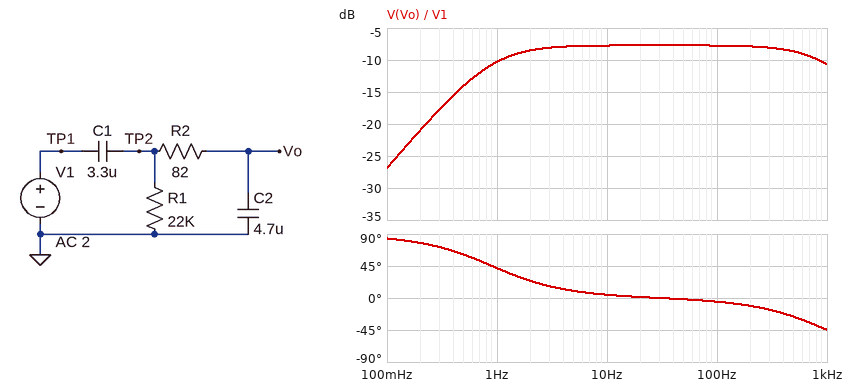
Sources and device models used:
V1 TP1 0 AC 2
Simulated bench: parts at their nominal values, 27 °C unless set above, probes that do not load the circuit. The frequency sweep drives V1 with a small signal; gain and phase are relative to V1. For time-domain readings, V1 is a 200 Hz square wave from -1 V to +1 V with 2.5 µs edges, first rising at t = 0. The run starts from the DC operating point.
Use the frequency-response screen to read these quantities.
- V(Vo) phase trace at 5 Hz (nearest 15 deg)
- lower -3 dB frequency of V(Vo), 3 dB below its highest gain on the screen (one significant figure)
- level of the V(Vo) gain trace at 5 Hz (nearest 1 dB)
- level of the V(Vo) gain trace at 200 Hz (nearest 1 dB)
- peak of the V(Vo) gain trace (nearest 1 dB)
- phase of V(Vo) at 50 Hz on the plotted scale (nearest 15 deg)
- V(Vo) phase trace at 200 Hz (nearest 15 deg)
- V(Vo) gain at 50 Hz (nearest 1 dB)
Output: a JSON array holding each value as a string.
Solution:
["15 deg", "900 mHz", "-8 dB", "-8 dB", "-8 dB", "0 deg", "-15 deg", "-8 dB"]
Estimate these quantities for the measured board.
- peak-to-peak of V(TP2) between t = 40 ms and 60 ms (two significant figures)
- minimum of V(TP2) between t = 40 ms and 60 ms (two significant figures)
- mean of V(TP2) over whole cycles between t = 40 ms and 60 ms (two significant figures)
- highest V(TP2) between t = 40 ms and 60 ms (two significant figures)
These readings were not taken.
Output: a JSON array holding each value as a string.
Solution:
["3.2 V", "-1.3 V", "310 mV", "1.9 V"]
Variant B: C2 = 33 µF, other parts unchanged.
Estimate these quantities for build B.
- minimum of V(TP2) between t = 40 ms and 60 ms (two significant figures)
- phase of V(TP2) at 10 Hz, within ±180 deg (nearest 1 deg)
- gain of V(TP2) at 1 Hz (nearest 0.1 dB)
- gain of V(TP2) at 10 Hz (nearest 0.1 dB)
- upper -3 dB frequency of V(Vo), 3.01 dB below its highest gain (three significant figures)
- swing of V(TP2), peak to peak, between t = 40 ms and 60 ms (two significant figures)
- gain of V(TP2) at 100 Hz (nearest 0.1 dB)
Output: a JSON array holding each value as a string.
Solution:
["-1.8 V", "10 deg", "-21.0 dB", "-20.7 dB", "649 Hz", "3.8 V", "-15.1 dB"]
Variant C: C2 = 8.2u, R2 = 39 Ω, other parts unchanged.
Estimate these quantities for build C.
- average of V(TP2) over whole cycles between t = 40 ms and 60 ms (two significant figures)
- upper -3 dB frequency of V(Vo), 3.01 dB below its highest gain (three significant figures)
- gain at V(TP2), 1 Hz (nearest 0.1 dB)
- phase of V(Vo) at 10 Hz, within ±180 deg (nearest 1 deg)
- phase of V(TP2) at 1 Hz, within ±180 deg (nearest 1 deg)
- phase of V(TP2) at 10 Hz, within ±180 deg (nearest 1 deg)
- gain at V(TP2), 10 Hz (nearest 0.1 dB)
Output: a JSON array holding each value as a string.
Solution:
["230 mV", "1.74 kHz", "-12.3 dB", "3 deg", "32 deg", "4 deg", "-10.9 dB"]
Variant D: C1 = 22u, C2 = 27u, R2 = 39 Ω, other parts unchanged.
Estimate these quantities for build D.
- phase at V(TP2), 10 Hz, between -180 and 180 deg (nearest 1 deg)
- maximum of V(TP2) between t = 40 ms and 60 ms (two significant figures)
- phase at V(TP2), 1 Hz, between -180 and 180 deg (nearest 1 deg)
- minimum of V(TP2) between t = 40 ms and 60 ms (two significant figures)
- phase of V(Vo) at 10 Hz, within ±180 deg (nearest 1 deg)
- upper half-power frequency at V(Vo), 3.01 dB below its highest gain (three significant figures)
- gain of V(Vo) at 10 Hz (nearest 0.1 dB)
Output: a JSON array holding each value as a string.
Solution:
["3 deg", "2.0 V", "9 deg", "-1.1 V", "-1 deg", "337 Hz", "-7.0 dB"]
